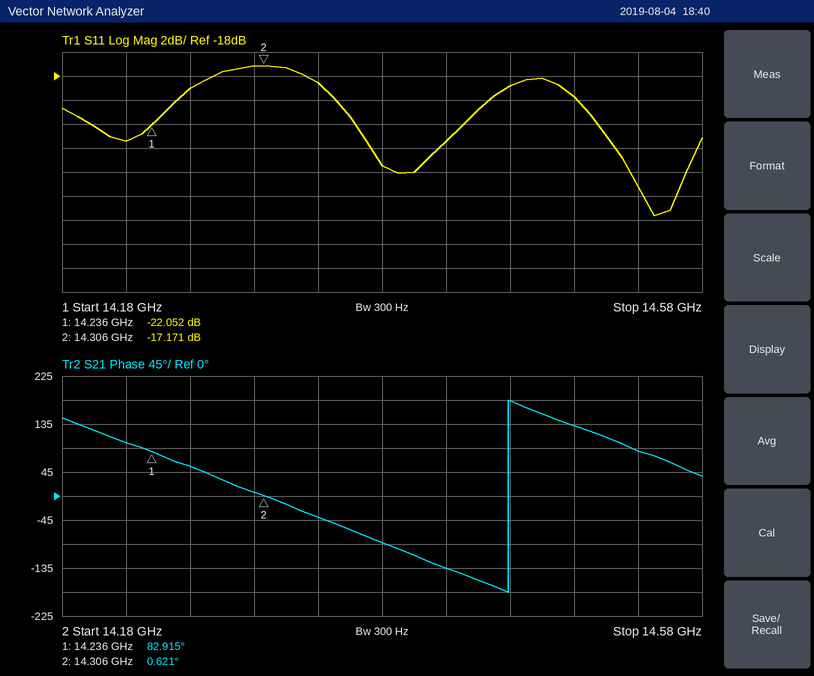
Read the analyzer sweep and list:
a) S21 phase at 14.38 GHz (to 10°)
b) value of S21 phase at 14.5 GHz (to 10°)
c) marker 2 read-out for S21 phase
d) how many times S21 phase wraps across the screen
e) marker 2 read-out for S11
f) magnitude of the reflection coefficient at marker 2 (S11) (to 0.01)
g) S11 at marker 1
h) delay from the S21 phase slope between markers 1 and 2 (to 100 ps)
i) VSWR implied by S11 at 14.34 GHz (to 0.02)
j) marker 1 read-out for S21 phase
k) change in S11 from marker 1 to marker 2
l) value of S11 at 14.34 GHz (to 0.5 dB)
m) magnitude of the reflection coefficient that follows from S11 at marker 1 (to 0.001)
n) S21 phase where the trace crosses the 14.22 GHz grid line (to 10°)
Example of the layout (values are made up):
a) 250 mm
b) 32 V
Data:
a) -90°
b) 130°
c) 0.621°
d) 1
e) -17.171 dB
f) 0.14
g) -22.052 dB
h) 3.3 ns
i) 1.26
j) 82.915°
k) 4.881 dB
l) -18.5 dB
m) 0.079
n) 100°
